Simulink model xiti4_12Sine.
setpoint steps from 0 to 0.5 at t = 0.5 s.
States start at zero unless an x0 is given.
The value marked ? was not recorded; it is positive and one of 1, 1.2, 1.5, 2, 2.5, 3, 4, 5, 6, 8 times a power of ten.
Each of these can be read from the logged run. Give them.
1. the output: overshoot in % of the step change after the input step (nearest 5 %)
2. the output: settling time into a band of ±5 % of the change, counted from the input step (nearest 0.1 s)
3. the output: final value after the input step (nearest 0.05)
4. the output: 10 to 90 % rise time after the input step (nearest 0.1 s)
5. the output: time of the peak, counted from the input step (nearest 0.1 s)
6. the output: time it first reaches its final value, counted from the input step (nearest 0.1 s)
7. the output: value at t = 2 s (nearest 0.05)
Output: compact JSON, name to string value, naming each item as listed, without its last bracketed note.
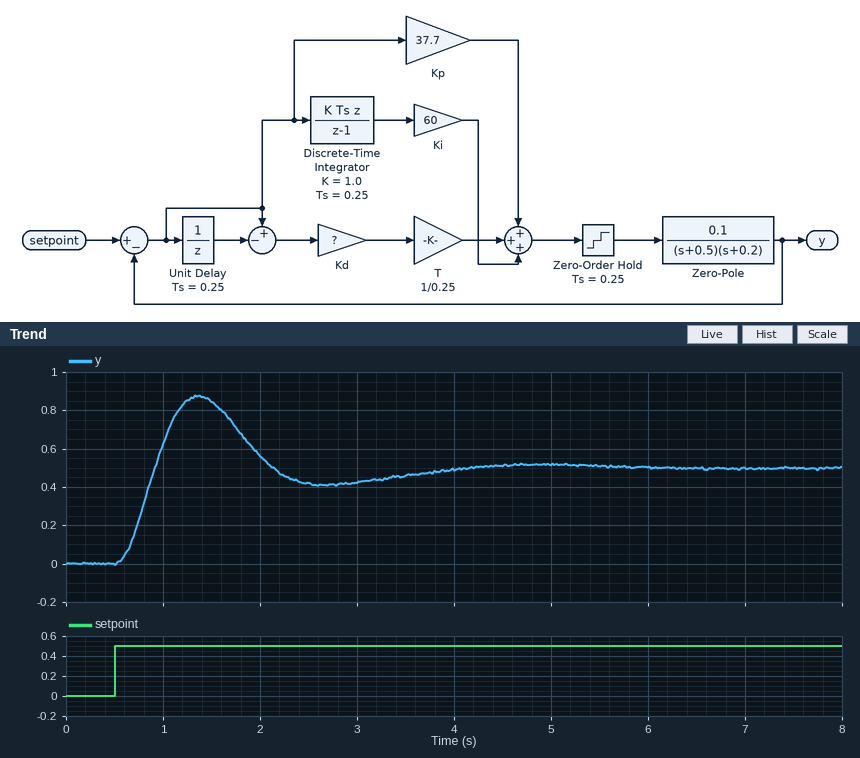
{"the output: overshoot in % of the step change after the input step": "75 %", "the output: settling time into a band of ±5 % of the change, counted from the input step": "3.2 s", "the output: final value after the input step": "0.50", "the output: 10 to 90 % rise time after the input step": "0.3 s", "the output: time of the peak, counted from the input step": "0.9 s", "the output: time it first reaches its final value, counted from the input step": "0.4 s", "the output: value at t = 2 s": "0.55"}
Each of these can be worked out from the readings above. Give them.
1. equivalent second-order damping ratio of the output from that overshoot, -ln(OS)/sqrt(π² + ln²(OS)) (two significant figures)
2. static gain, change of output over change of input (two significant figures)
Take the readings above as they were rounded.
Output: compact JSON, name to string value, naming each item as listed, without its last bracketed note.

{"equivalent second-order damping ratio of the output from that overshoot, -ln(OS)/sqrt(π² + ln²(OS))": "0.091", "static gain, change of output over change of input": "1.0"}
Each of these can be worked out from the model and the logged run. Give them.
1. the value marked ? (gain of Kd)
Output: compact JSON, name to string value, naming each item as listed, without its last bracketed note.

{"the value marked ?": "25"}
